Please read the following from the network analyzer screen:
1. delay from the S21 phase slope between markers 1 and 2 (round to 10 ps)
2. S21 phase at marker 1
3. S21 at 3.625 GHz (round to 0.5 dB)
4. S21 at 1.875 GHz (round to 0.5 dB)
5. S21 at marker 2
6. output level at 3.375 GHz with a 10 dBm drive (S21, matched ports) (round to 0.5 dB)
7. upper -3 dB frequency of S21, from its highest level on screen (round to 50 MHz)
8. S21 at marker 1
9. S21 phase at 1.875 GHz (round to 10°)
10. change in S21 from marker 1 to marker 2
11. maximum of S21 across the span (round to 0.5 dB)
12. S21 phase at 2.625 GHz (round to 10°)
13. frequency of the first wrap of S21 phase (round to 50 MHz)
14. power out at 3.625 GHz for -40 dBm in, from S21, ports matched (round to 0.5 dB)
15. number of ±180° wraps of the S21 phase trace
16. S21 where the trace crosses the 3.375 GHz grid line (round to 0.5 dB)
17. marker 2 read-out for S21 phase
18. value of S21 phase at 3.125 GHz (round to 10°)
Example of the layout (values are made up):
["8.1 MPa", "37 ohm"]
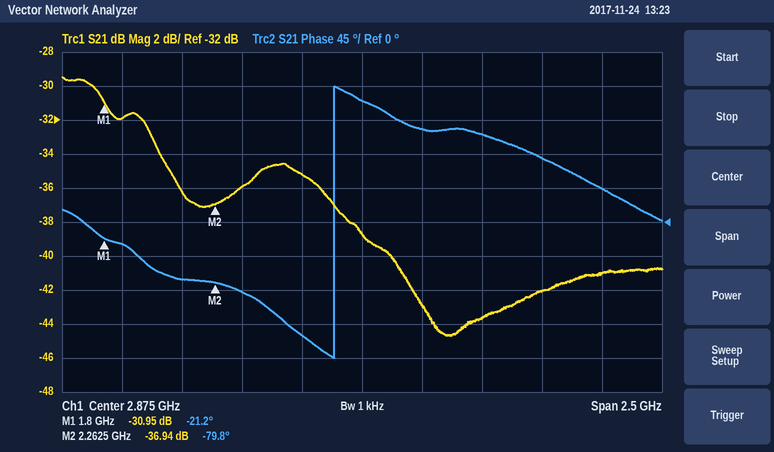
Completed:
["350 ps", "-21.2°", "-42.0 dB", "-32.0 dB", "-36.94 dB", "-33.5 dBm", "2.00 GHz", "-30.95 dB", "-30°", "-5.99 dB", "-29.5 dB", "-150°", "2.75 GHz", "-82.0 dBm", "1", "-43.5 dB", "-79.8°", "120°"]
